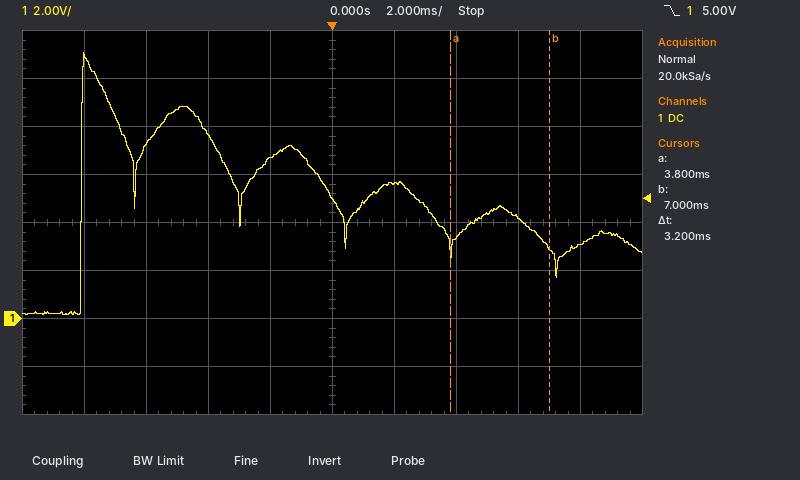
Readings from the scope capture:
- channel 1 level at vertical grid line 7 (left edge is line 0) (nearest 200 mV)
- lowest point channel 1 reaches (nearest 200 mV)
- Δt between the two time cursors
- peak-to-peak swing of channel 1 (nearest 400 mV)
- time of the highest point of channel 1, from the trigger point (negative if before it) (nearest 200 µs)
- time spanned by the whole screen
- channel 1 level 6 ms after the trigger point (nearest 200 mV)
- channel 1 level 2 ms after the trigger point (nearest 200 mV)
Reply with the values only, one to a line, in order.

3.4 V
200 mV
3.2 ms
10.8 V
-8.0 ms
20 ms
4.2 V
5.6 V
